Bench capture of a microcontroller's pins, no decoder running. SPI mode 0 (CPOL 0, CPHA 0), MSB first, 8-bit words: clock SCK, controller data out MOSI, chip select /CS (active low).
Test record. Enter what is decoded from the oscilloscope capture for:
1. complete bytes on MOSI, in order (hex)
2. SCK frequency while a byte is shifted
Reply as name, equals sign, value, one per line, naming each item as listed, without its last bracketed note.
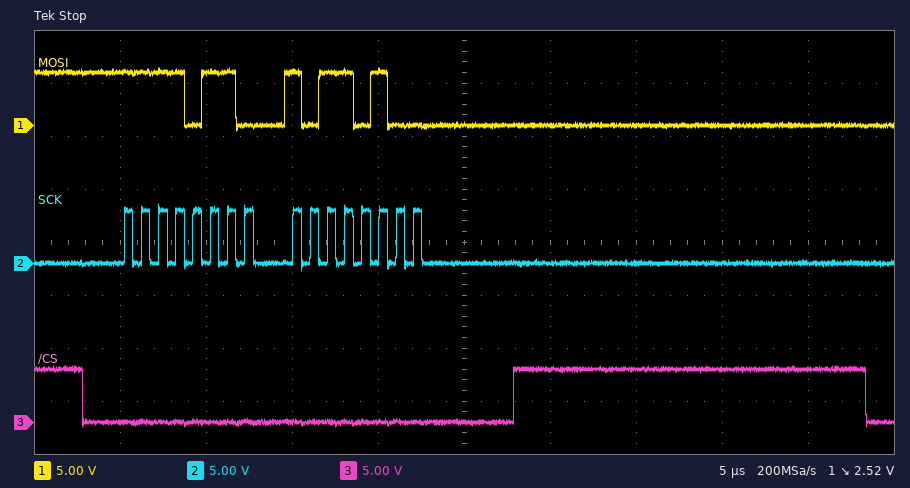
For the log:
complete bytes on MOSI, in order = F6 B4
SCK frequency while a byte is shifted = 1 MHz
